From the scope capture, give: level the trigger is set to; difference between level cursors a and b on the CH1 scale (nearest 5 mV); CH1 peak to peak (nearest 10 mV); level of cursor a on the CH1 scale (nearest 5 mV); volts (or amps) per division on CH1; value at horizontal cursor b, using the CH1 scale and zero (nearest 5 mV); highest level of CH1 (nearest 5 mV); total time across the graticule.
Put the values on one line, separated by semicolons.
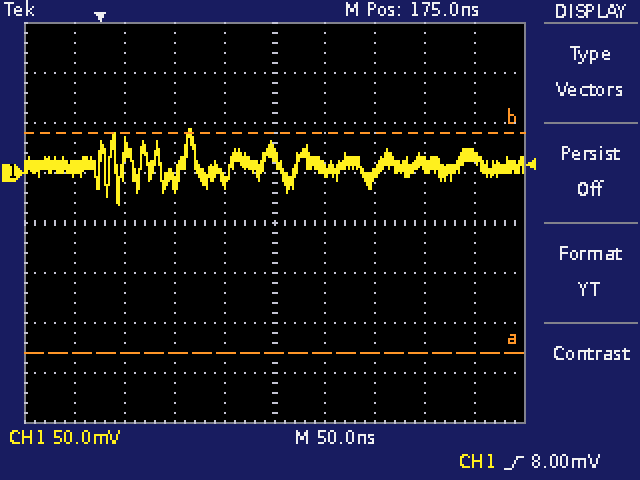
8.00 mV; 220 mV; 80 mV; -180 mV; 50 mV; 40 mV; 45 mV; 500 ns
